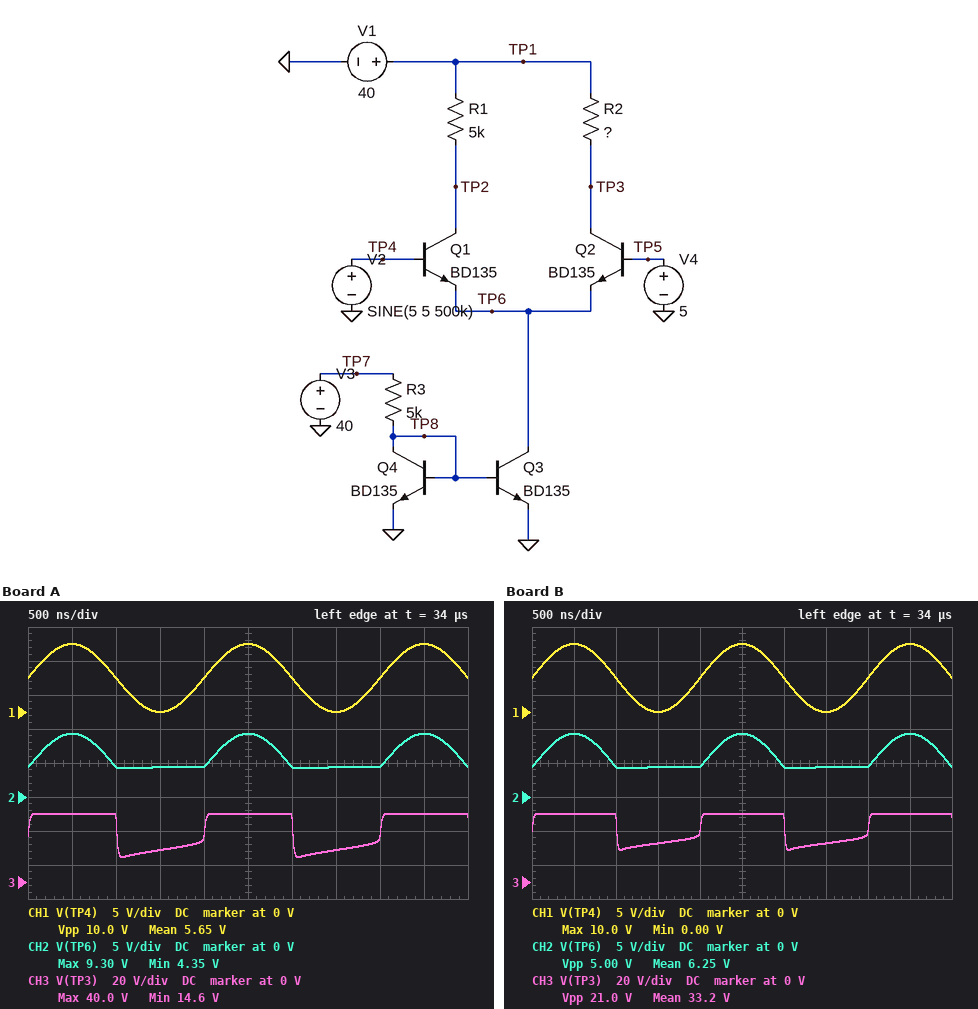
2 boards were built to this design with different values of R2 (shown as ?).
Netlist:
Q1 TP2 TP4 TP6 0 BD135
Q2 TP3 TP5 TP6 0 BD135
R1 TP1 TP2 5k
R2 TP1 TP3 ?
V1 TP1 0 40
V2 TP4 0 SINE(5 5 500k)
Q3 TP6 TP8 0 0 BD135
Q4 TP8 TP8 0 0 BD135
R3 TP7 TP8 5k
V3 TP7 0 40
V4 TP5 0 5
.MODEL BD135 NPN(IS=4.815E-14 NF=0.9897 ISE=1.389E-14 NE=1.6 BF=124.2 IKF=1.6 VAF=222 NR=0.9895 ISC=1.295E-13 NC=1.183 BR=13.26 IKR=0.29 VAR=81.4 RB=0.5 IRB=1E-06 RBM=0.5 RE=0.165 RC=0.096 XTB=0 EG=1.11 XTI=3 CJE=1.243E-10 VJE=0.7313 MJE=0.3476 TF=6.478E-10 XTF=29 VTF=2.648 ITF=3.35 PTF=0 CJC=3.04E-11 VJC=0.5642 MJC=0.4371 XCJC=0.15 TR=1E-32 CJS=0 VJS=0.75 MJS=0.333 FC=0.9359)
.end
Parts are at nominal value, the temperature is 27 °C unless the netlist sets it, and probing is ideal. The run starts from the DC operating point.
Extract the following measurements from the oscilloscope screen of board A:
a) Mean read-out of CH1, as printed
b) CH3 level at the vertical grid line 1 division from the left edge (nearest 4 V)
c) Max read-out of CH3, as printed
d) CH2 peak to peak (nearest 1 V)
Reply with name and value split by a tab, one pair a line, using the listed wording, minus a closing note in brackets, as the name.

Mean read-out of CH1, as printed	5.65 V
CH3 level at the vertical grid line 1 division from the left edge	40 V
Max read-out of CH3, as printed	40.0 V
CH2 peak to peak	5 V
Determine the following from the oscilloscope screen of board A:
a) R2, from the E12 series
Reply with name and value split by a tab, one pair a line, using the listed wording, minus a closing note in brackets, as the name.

R2, from the E12 series	2.7 kΩ
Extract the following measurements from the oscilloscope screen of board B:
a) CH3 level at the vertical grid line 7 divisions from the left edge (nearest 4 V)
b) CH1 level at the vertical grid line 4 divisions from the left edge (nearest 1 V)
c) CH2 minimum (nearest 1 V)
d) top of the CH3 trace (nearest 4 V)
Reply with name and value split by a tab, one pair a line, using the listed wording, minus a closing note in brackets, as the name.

CH3 level at the vertical grid line 7 divisions from the left edge	24 V
CH1 level at the vertical grid line 4 divisions from the left edge	5 V
CH2 minimum	4 V
top of the CH3 trace	40 V
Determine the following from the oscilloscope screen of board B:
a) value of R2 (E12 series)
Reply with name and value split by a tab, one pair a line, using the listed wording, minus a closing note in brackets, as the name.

value of R2	2.2 kΩ
